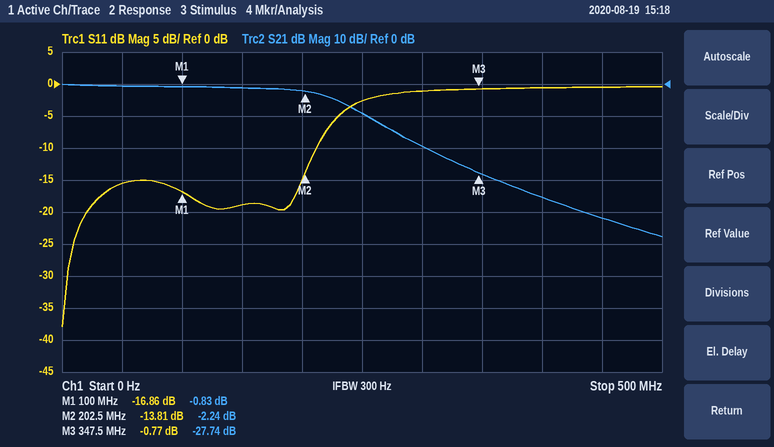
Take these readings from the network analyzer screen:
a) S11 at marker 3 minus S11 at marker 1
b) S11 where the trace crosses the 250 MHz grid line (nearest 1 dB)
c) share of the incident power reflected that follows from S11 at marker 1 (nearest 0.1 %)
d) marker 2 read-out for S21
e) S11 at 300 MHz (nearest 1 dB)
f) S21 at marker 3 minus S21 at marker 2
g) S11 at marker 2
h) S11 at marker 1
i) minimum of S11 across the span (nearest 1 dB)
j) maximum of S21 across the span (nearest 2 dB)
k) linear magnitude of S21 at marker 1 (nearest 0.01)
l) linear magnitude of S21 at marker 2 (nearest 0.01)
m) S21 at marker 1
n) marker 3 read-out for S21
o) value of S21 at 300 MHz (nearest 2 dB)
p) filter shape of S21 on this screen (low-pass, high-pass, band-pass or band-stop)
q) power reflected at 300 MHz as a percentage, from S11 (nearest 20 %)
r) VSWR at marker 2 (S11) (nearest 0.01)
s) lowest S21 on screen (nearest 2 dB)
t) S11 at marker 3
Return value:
16.09 dB
-3 dB
2.1 %
-2.24 dB
-1 dB
-25.50 dB
-13.81 dB
-16.86 dB
-38 dB
0 dB
0.91
0.77
-0.83 dB
-27.74 dB
-20 dB
low-pass
80 %
1.51
-48 dB
-0.77 dB
